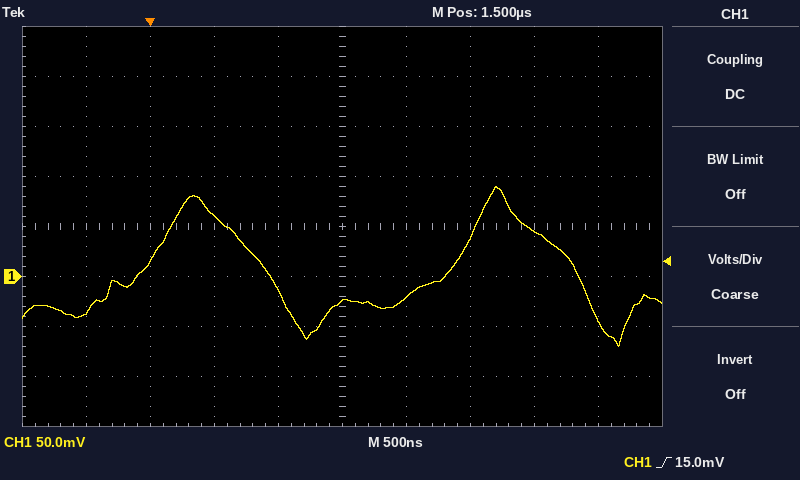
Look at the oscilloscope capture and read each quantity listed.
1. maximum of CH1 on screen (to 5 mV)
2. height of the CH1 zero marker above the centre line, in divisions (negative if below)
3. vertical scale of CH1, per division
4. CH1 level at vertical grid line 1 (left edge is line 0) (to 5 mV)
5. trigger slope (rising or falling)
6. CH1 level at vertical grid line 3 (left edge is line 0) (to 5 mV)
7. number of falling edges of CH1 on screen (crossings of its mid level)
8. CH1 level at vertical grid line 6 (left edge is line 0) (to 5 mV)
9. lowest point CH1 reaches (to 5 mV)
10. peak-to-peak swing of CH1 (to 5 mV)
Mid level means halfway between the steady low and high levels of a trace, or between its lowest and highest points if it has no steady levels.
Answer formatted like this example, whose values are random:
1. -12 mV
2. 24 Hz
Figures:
1. 90 mV
2. -1.0 div
3. 50 mV
4. -35 mV
5. rising
6. 60 mV
7. 2
8. -20 mV
9. -70 mV
10. 160 mV
